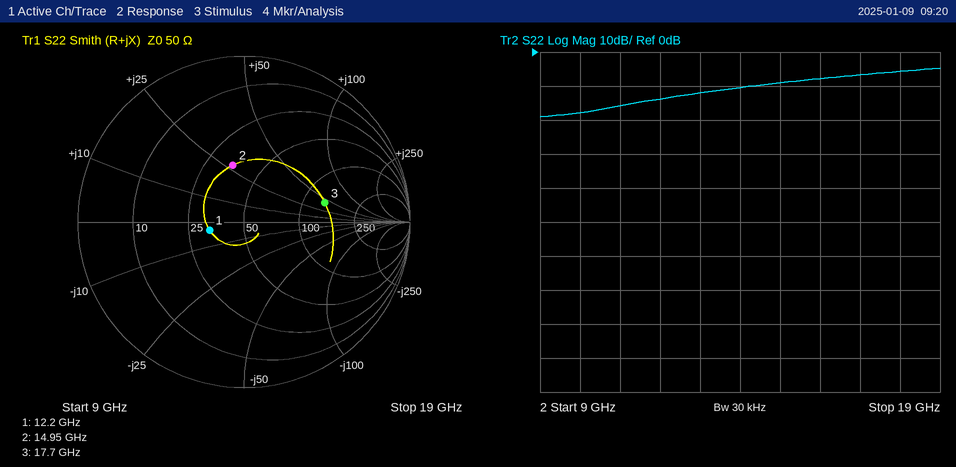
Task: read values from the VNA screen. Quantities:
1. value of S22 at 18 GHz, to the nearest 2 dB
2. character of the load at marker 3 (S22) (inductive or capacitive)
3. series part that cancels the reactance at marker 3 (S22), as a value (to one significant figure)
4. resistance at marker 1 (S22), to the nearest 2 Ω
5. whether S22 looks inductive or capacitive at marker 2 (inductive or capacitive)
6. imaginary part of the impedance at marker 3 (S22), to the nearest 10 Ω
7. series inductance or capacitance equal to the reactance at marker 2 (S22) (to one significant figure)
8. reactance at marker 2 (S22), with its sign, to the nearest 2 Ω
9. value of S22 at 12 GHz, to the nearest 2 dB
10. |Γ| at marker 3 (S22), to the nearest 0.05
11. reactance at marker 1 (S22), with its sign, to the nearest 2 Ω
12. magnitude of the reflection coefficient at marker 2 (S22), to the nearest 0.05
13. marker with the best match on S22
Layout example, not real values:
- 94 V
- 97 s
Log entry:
- -6 dB
- inductive
- 200 fF
- 32 Ω
- inductive
- +40 Ω
- 300 pH
- +28 Ω
- -14 dB
- 0.50
- -4 Ω
- 0.35
- marker 1
